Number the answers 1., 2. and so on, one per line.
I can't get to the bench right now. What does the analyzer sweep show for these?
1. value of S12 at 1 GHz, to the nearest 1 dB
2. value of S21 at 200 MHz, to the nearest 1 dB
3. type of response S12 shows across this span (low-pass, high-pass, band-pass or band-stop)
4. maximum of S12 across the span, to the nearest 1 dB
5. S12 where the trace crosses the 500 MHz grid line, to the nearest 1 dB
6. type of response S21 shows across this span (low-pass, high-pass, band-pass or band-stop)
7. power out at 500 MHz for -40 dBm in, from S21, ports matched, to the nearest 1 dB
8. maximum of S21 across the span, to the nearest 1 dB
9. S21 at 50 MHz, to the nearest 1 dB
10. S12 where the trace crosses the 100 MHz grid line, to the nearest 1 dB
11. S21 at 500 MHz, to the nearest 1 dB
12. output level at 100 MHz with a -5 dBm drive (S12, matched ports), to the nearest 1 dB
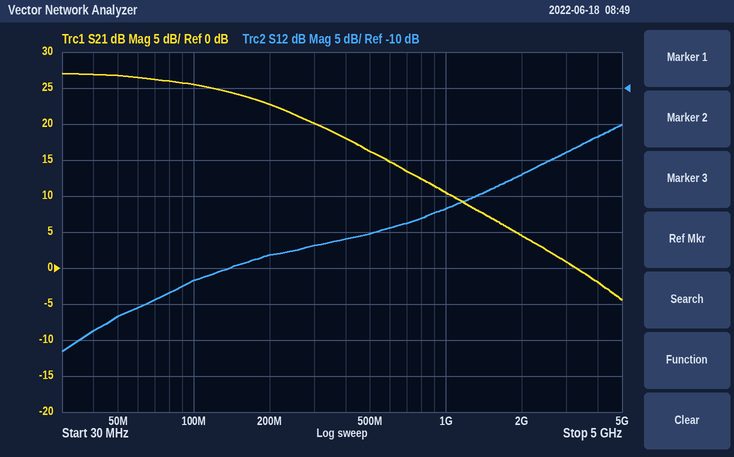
1. -27 dB
2. 23 dB
3. high-pass
4. -15 dB
5. -30 dB
6. low-pass
7. -24 dBm
8. 27 dB
9. 27 dB
10. -37 dB
11. 16 dB
12. -42 dBm
